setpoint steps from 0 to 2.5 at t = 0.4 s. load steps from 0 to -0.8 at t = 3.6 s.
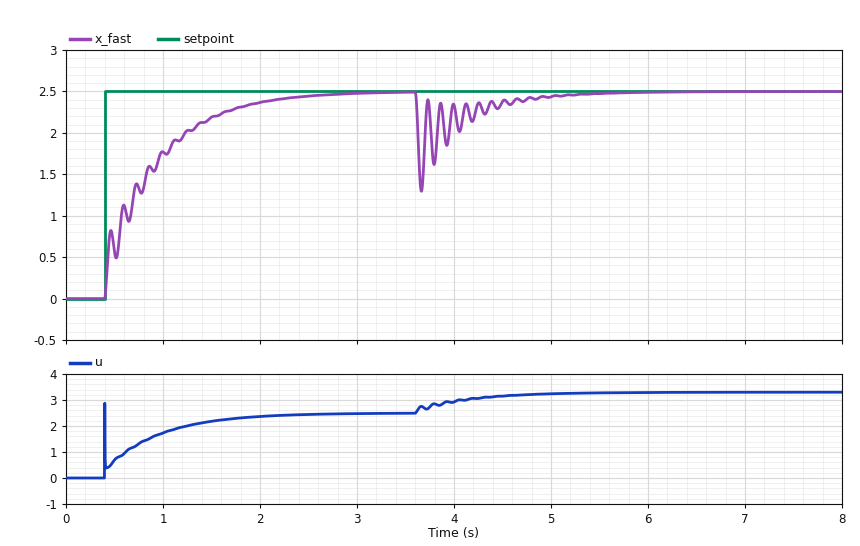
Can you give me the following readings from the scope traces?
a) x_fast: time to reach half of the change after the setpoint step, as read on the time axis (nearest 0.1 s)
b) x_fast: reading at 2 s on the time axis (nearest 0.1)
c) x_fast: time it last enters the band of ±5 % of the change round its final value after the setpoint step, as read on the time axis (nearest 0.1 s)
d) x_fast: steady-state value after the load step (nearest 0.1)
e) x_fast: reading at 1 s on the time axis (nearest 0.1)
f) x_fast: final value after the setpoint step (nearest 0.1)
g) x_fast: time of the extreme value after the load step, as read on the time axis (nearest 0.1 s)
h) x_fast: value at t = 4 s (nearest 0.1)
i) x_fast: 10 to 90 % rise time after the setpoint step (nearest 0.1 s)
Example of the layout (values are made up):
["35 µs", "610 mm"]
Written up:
["0.7 s", "2.4", "2.0 s", "2.5", "1.8", "2.5", "3.7 s", "2.3", "1.2 s"]
